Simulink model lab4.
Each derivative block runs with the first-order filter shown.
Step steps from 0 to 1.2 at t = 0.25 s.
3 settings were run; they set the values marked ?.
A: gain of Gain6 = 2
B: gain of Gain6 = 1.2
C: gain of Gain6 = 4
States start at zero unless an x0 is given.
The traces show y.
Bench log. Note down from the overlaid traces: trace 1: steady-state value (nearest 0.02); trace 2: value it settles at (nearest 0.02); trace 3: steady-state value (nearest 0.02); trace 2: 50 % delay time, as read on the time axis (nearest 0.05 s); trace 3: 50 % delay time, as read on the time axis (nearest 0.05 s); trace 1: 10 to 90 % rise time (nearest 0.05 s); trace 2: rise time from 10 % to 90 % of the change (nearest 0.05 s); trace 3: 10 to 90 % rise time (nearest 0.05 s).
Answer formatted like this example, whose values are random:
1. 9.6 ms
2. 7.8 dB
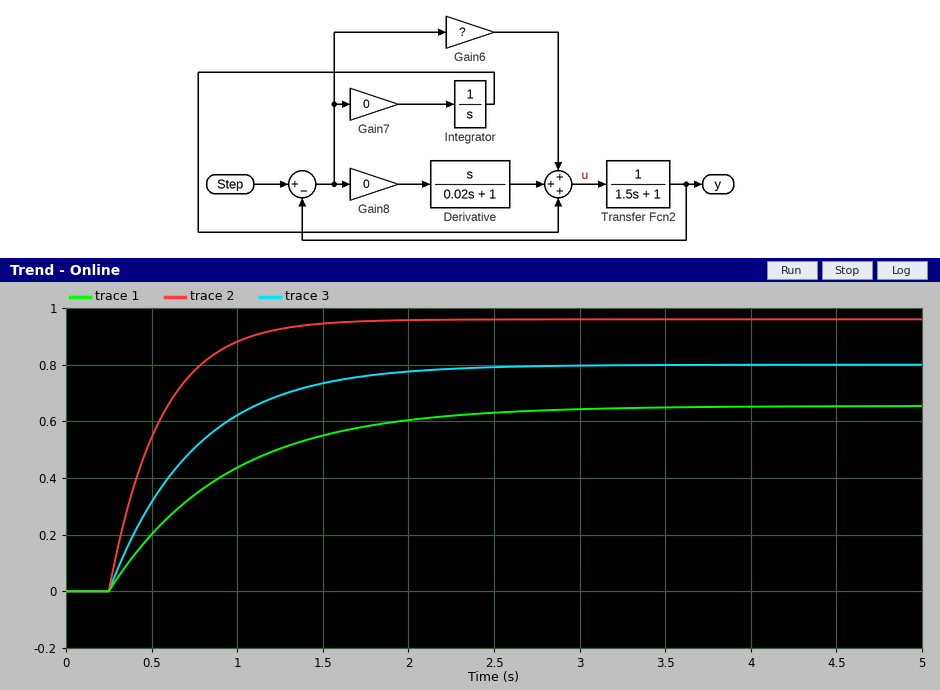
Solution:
1. 0.66
2. 0.96
3. 0.80
4. 0.45 s
5. 0.60 s
6. 1.50 s
7. 0.65 s
8. 1.10 s
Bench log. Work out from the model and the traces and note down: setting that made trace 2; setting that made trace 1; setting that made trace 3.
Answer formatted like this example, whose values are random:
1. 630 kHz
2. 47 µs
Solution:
1. C
2. B
3. A
